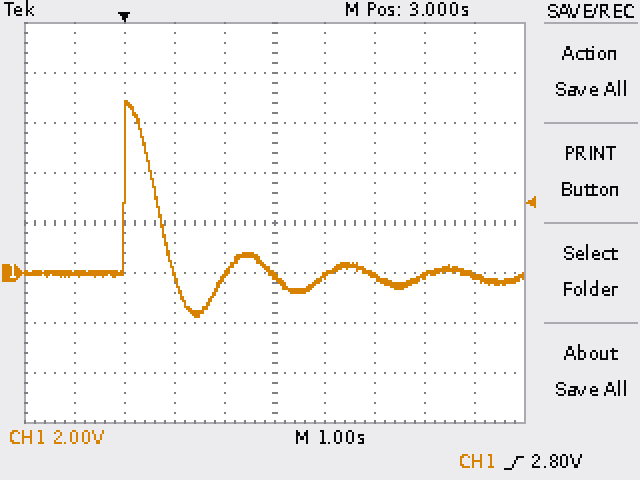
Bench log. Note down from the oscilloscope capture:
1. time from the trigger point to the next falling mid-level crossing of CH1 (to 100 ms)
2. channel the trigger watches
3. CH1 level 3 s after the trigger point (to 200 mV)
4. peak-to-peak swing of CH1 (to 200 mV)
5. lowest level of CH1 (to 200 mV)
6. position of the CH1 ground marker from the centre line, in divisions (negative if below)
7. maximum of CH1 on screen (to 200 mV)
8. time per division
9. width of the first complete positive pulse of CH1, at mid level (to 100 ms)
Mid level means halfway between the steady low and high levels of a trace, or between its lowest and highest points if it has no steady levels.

700 ms
CH1
-200 mV
8.6 V
-1.8 V
-1.0 div
6.8 V
1 s
700 ms
